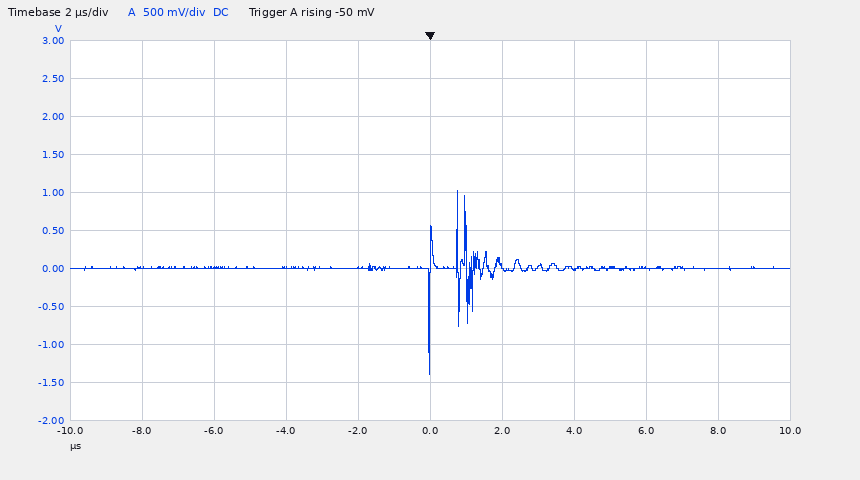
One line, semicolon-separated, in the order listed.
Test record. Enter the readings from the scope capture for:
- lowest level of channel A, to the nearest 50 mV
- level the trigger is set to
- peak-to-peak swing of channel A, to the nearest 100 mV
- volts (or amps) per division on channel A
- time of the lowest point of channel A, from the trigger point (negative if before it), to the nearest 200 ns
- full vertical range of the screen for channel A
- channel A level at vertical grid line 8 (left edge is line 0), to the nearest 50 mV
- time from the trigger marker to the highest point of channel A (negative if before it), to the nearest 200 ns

-1.40 V; -50 mV; 2.40 V; 500 mV; 0.0 µs; 5 V; 0 mV; +800 ns
